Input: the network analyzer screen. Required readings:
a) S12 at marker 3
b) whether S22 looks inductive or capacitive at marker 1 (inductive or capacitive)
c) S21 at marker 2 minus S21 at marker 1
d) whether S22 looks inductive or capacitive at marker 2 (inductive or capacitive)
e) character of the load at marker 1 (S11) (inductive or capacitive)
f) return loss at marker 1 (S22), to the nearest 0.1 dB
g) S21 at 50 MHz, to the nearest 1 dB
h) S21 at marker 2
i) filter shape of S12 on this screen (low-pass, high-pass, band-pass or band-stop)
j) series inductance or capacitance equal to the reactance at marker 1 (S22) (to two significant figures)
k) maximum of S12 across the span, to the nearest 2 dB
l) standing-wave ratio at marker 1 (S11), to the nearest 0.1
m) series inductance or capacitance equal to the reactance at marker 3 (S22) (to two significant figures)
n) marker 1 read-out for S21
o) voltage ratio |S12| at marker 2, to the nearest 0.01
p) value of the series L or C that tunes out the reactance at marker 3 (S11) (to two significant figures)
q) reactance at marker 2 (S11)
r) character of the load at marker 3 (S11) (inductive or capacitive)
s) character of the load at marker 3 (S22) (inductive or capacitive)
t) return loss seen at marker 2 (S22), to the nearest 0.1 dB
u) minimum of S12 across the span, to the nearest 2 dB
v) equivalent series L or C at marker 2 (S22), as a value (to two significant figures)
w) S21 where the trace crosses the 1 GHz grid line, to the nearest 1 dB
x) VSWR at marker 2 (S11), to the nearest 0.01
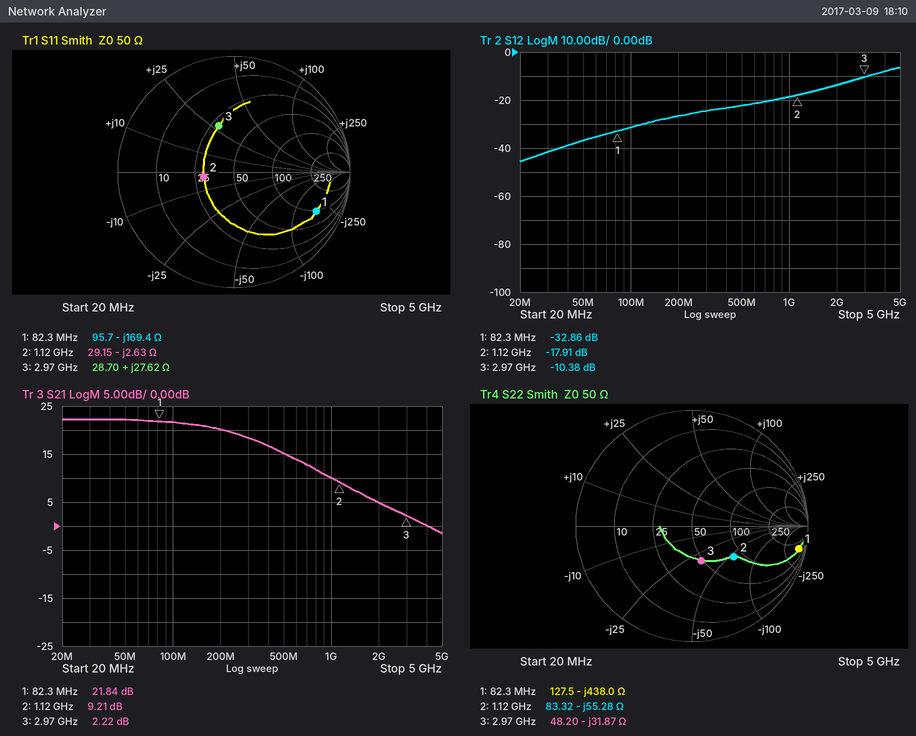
-10.38 dB
capacitive
-12.63 dB
capacitive
capacitive
0.5 dB
22 dB
9.21 dB
high-pass
4.4 pF
-6 dB
8.3
1.7 pF
21.84 dB
0.13
1.9 pF
-2.63 Ω
inductive
capacitive
7.0 dB
-46 dB
2.6 pF
10 dB
1.72
